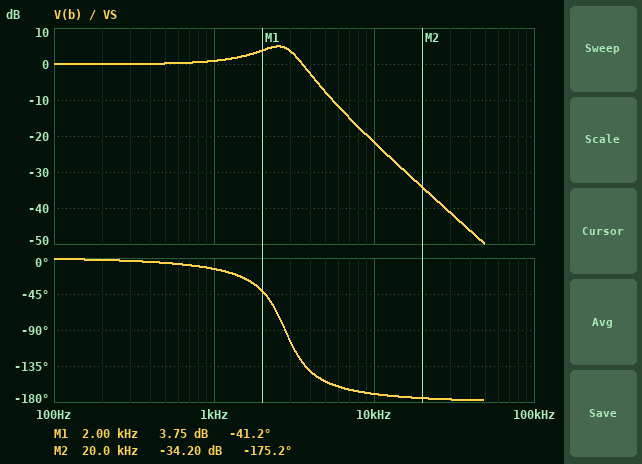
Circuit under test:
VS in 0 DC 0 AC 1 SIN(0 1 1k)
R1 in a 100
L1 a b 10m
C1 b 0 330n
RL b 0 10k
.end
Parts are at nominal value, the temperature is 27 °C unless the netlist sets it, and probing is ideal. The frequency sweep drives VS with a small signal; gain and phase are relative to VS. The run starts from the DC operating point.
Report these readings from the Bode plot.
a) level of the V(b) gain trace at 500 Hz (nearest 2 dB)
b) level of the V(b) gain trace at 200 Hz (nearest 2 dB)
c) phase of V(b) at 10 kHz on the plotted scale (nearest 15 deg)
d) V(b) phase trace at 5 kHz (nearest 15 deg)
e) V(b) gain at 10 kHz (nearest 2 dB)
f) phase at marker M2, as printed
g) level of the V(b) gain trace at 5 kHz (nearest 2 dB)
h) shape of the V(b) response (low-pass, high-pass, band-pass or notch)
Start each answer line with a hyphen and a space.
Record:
- 0 dB
- 0 dB
- -165 deg
- -150 deg
- -22 dB
- -175.2 deg
- -8 dB
- low-pass
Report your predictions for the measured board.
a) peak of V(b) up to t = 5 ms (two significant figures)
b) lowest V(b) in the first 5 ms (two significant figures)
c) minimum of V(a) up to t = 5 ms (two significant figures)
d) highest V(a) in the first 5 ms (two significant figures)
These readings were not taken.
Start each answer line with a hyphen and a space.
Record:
- 1.2 V
- -1.1 V
- -960 mV
- 960 mV
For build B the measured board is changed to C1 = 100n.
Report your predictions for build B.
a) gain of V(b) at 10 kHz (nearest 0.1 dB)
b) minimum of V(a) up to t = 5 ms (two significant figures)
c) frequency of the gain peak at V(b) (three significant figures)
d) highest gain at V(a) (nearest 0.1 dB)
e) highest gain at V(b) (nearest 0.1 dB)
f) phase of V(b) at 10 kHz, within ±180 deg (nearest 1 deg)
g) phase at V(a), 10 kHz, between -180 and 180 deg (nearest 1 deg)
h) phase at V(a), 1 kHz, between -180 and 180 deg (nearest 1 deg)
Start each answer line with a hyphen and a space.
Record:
- -9.6 dB
- -990 mV
- 4.90 kHz
- 0 dB
- 9.3 dB
- -167 deg
- 12 deg
- -4 deg
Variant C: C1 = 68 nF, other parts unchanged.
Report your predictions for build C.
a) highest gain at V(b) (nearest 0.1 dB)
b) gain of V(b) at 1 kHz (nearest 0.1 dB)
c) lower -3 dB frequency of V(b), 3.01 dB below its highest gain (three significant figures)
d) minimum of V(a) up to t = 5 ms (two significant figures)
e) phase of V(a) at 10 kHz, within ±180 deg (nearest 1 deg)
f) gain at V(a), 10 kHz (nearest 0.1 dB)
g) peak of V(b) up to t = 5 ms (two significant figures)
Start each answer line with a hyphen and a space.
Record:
- 10.5 dB
- 0.1 dB
- 4.99 kHz
- -990 mV
- 14 deg
- -0.3 dB
- 1.0 V
